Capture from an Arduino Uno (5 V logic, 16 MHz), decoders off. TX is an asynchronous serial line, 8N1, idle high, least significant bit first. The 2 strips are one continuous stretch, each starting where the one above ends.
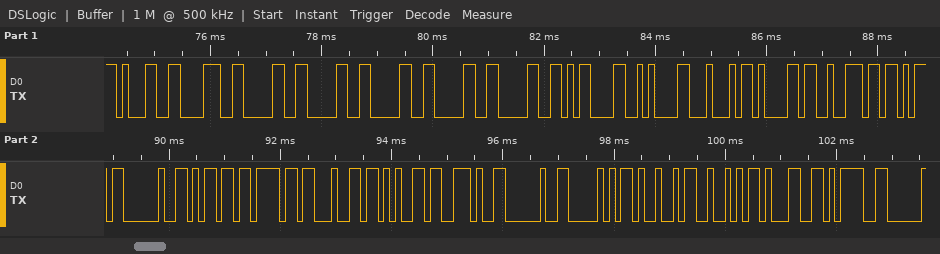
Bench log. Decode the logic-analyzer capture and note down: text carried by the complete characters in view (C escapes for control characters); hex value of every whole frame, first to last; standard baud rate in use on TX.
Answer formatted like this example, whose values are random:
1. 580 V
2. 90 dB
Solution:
1. "1800000\r\nDark mode. PIR1="
2. 31 38 30 30 30 30 30 0D 0A 44 61 72 6B 20 6D 6F 64 65 2E 20 50 49 52 31 3D
3. 9600 baud
